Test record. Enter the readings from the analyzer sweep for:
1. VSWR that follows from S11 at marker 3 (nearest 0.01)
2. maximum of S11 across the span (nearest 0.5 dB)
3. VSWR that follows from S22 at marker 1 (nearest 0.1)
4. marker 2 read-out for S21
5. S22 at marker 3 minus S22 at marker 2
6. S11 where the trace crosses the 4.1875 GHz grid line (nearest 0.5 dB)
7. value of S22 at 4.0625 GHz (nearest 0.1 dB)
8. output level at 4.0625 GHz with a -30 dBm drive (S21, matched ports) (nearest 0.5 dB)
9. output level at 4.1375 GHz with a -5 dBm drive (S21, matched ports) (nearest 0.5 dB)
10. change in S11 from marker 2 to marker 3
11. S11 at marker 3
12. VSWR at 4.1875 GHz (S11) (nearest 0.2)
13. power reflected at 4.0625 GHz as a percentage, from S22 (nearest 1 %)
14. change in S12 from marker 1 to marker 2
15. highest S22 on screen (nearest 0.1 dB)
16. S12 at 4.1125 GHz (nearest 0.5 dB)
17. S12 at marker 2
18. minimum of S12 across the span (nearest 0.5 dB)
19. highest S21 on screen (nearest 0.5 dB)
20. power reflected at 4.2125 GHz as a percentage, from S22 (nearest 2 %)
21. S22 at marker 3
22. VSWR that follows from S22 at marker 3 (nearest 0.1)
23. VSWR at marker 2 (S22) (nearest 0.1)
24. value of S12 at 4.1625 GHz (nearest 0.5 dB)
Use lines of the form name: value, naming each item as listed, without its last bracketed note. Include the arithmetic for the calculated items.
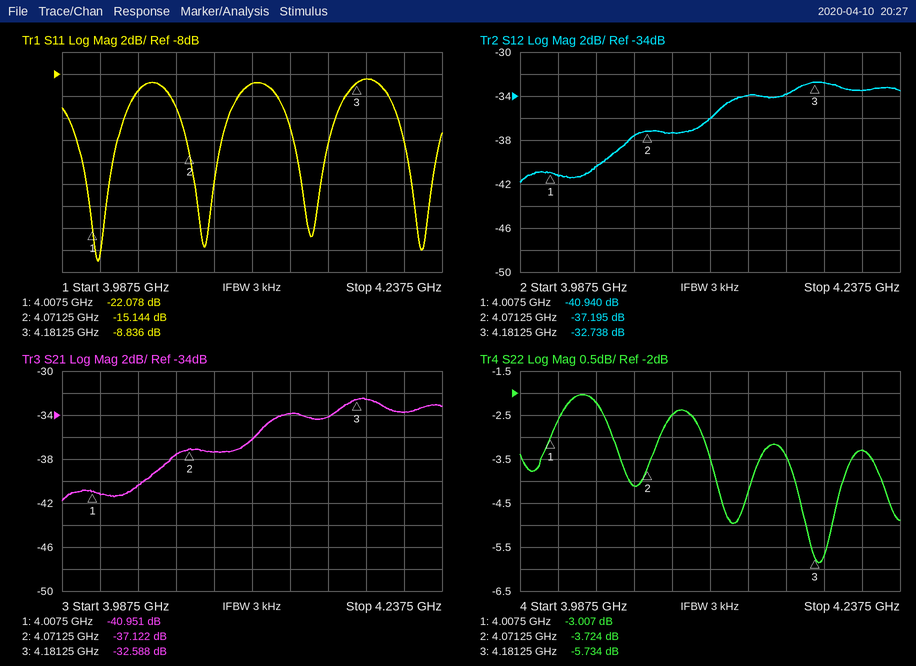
VSWR that follows from S11 at marker 3: (1 + 0.3616)/(1 − 0.3616) ≈ 2.13
maximum of S11 across the span: -8.5 dB
VSWR that follows from S22 at marker 1: (1 + 0.7074)/(1 − 0.7074) ≈ 5.8
marker 2 read-out for S21: -37.122 dB
S22 at marker 3 minus S22 at marker 2: -5.734 − (-3.724) = -2.010 dB
S11 where the trace crosses the 4.1875 GHz grid line: -8.5 dB
value of S22 at 4.0625 GHz: -4.1 dB
output level at 4.0625 GHz with a -30 dBm drive (S21, matched ports): -30 dBm + (-37.5 dB) = -67.5 dBm
output level at 4.1375 GHz with a -5 dBm drive (S21, matched ports): -5 dBm + (-34.0 dB) = -39.0 dBm
change in S11 from marker 2 to marker 3: -8.836 − (-15.144) = 6.308 dB
S11 at marker 3: -8.836 dB
VSWR at 4.1875 GHz (S11): |Γ| = 10^(-8.5/20) = 0.3758; VSWR = (1 + 0.3758)/(1 − 0.3758) ≈ 2.2
power reflected at 4.0625 GHz as a percentage, from S22: 10^(-4.1/10) ≈ 39 %
change in S12 from marker 1 to marker 2: -37.195 − (-40.94) = 3.745 dB
highest S22 on screen: -2.0 dB
S12 at 4.1125 GHz: -36.0 dB
S12 at marker 2: -37.195 dB
minimum of S12 across the span: -42.0 dB
highest S21 on screen: -32.5 dB
power reflected at 4.2125 GHz as a percentage, from S22: 10^(-3.3/10) ≈ 46.8 %, so 46 % to the nearest 2 %
S22 at marker 3: -5.734 dB
VSWR that follows from S22 at marker 3: (1 + 0.5168)/(1 − 0.5168) ≈ 3.1
VSWR at marker 2 (S22): (1 + 0.6513)/(1 − 0.6513) ≈ 4.7
value of S12 at 4.1625 GHz: -34.0 dB
